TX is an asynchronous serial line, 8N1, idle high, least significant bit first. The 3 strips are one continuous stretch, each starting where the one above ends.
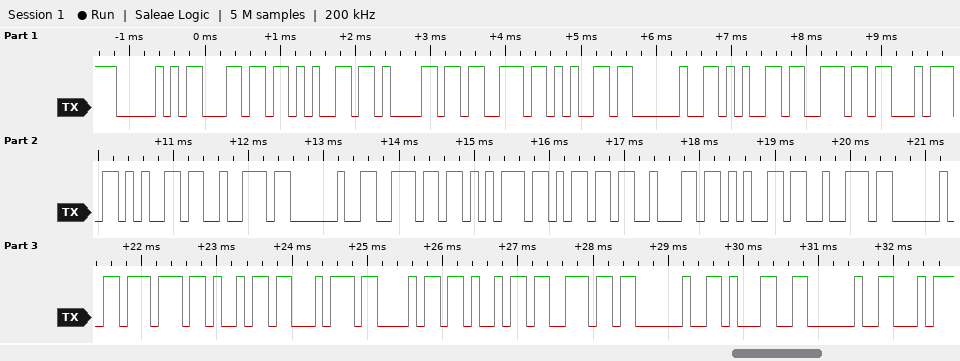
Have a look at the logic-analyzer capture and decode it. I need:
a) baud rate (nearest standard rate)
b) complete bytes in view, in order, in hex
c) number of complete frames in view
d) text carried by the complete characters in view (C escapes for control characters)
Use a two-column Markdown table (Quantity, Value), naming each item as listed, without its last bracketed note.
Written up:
| Quantity | Value |
|---|---|
| baud rate | 9600 baud |
| complete bytes in view, in order, in hex | 50 6C 65 61 73 65 20 65 6E 74 65 72 20 6E 75 6D 62 65 72 20 77 69 74 68 69 6E 20 31 20 |
| number of complete frames in view | 29 |
| text carried by the complete characters in view | "Please enter number within 1 " |
